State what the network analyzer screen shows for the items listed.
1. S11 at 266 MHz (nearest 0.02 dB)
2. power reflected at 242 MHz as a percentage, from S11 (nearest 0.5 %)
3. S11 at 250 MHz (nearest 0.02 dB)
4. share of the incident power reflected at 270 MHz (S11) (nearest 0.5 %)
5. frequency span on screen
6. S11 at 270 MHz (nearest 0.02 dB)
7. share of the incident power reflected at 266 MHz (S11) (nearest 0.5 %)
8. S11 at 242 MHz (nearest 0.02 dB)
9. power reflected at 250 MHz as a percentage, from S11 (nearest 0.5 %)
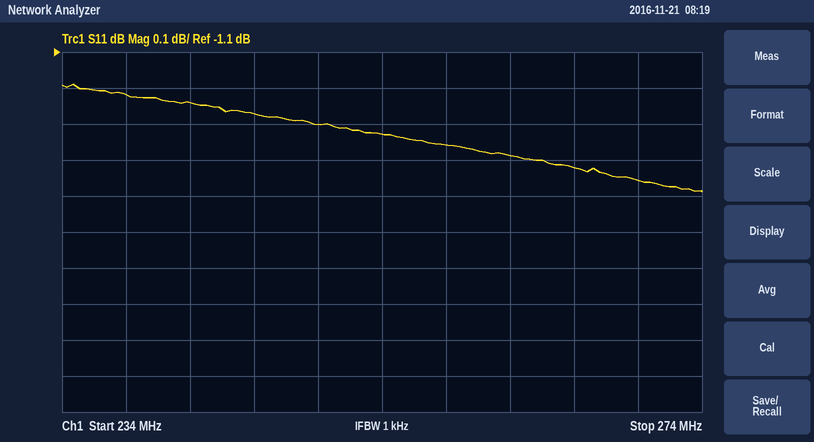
-1.42 dB
75.0 %
-1.30 dB
71.5 %
40 MHz
-1.46 dB
72.0 %
-1.24 dB
74.0 %
